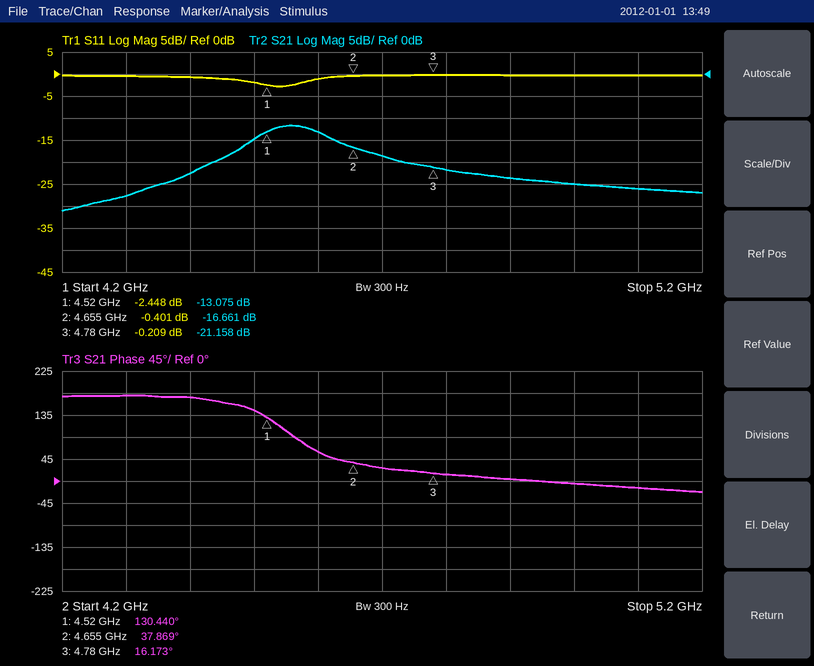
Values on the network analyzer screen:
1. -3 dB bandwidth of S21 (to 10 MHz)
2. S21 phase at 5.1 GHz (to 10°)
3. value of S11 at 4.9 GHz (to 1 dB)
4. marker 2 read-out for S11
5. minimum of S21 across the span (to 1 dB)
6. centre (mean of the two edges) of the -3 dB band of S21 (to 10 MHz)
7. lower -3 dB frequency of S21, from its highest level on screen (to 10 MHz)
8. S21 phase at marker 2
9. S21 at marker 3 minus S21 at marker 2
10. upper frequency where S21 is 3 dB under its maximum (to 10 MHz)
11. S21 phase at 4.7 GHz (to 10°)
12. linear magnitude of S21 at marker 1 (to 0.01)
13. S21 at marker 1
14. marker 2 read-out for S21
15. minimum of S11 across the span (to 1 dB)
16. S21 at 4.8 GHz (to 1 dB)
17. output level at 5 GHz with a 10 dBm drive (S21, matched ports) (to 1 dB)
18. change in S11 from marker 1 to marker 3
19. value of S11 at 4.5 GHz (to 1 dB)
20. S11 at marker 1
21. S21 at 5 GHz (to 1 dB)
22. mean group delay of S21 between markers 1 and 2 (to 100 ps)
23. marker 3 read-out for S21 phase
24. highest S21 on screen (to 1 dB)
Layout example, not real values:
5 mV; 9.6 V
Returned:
120 MHz; -10°; 0 dB; -0.401 dB; -31 dB; 4.56 GHz; 4.50 GHz; 37.869°; -4.497 dB; 4.62 GHz; 30°; 0.22; -13.075 dB; -16.661 dB; -3 dB; -22 dB; -15 dBm; 2.239 dB; -2 dB; -2.448 dB; -25 dB; 1.9 ns; 16.173°; -12 dB
